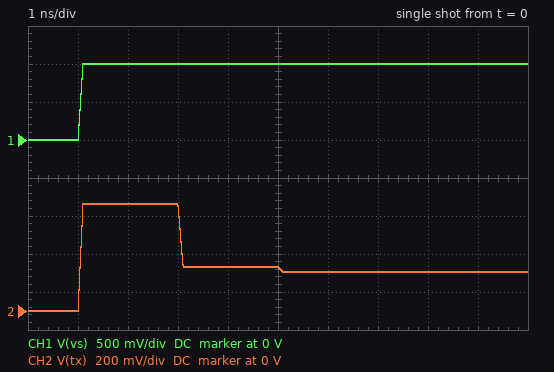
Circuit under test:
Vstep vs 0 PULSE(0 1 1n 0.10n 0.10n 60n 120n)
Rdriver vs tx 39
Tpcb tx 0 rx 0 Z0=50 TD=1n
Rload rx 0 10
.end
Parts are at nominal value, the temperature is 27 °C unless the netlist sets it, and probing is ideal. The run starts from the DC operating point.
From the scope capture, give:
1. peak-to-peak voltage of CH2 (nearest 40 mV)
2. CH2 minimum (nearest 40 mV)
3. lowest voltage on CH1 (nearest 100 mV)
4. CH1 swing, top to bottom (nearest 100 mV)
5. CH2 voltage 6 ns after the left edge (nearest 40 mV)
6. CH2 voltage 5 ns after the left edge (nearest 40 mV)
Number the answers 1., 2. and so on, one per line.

1. 560 mV
2. 0 V
3. 0 V
4. 1.0 V
5. 200 mV
6. 240 mV
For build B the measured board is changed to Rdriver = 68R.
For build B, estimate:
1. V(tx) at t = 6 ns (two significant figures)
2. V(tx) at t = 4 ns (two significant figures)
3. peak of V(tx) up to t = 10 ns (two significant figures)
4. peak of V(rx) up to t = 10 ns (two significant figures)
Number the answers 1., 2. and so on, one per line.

1. 130 mV
2. 98 mV
3. 420 mV
4. 140 mV
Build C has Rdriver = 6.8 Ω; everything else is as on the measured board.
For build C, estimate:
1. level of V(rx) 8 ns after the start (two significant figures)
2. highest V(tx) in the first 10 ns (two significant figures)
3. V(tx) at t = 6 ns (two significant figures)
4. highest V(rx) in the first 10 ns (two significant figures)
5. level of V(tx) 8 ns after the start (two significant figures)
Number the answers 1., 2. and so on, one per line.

1. 520 mV
2. 880 mV
3. 670 mV
4. 560 mV
5. 630 mV
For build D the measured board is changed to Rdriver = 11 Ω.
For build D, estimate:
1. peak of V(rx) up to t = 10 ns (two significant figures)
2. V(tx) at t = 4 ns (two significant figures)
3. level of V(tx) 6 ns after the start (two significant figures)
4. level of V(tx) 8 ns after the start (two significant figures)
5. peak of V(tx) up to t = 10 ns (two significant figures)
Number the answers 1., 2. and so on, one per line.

1. 460 mV
2. 620 mV
3. 540 mV
4. 500 mV
5. 820 mV
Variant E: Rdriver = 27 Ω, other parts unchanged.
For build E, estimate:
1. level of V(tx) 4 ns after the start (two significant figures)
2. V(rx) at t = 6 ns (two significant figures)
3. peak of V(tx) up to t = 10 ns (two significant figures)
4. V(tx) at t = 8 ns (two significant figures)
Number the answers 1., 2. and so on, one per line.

1. 350 mV
2. 260 mV
3. 650 mV
4. 270 mV
